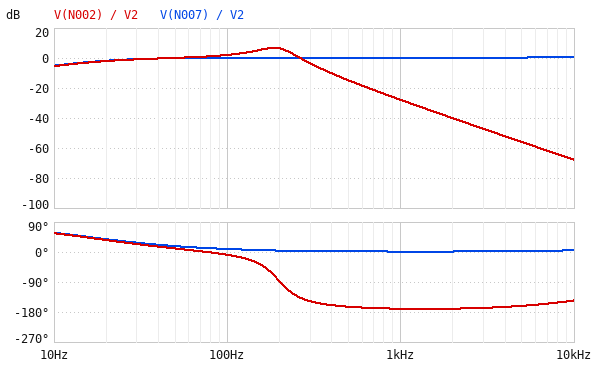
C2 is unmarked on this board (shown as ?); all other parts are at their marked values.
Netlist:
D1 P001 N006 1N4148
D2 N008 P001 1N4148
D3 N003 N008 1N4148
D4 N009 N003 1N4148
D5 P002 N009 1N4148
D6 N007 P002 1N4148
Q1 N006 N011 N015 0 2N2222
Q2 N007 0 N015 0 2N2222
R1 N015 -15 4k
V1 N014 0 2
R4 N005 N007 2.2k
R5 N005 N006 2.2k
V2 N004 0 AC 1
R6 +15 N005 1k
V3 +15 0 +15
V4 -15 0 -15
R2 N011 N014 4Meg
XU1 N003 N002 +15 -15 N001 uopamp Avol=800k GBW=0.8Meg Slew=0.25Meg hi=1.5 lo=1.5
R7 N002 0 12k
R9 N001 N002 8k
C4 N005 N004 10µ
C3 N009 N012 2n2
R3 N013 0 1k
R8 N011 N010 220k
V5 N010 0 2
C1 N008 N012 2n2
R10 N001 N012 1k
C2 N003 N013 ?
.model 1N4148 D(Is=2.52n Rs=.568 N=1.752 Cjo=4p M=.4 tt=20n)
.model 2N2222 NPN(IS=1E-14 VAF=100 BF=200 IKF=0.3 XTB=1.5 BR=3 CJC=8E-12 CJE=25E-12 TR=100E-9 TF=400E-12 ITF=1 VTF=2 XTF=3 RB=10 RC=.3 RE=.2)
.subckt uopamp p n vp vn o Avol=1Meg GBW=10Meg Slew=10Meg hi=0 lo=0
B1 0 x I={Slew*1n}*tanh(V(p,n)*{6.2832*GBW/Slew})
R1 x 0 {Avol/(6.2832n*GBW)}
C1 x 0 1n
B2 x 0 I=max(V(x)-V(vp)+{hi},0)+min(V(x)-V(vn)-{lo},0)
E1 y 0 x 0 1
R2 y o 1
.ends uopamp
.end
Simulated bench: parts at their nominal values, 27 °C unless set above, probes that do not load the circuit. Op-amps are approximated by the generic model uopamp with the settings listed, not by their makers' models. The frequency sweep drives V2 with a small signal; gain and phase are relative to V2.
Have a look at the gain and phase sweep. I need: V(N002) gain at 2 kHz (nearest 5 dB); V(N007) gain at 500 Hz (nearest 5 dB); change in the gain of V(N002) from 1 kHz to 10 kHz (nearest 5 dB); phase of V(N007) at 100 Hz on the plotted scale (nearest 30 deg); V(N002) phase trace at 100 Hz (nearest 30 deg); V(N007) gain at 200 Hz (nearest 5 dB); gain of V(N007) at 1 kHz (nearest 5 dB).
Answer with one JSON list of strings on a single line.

["-40 dB", "0 dB", "-40 dB", "0 deg", "0 deg", "0 dB", "0 dB"]
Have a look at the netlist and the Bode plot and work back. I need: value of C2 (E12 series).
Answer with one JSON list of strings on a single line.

["2.7 nF"]
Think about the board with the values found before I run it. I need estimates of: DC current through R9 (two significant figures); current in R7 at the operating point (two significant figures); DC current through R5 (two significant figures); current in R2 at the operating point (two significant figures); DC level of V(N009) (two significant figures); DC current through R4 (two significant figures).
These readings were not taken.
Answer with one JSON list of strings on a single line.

["630 µA", "630 µA", "2.0 mA", "500 nA", "7.7 V", "1.5 mA"]
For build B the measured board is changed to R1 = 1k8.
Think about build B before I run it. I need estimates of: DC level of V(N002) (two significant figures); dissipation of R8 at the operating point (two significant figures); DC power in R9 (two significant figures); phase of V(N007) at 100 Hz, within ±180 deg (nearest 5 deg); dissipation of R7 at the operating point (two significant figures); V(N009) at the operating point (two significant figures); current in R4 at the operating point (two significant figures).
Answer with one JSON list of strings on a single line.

["1.7 V", "19 µW", "170 µW", "15 deg", "250 µW", "920 mV", "4.3 mA"]
